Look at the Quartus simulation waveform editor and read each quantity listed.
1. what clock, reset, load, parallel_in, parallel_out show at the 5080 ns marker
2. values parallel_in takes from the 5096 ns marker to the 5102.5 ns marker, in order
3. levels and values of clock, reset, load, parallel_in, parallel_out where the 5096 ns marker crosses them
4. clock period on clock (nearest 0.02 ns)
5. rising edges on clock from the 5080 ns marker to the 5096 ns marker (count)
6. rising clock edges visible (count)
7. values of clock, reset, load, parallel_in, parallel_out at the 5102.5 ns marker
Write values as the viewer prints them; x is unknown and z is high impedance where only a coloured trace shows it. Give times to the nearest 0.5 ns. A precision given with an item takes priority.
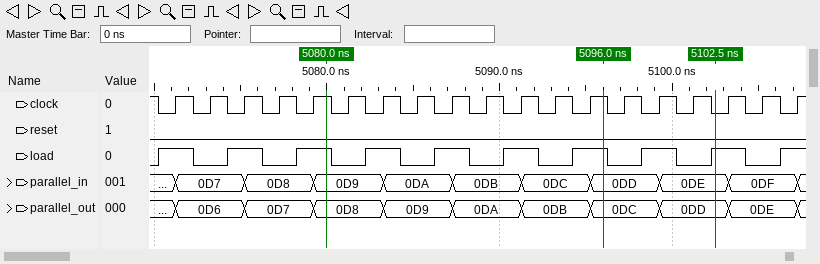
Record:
clock=1, reset=0, load=1, parallel_in=0D9, parallel_out=0D8
0DD, 0DE
clock=1, reset=0, load=1, parallel_in=0DD, parallel_out=0DC
2 ns
8
19
clock=0, reset=0, load=1, parallel_in=0DE, parallel_out=0DD
